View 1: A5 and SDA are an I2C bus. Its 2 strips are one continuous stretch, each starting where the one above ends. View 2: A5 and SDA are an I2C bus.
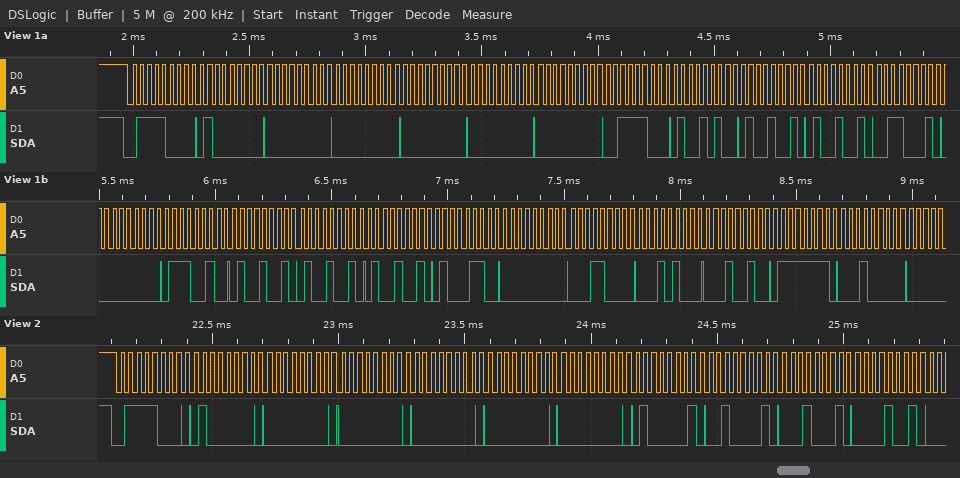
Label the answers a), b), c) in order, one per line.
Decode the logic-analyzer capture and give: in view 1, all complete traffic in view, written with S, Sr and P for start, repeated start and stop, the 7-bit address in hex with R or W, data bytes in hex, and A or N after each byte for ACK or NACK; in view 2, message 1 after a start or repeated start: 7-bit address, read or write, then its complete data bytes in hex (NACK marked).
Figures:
a) S 3CW A 40 A 00 A 00 A 00 A 00 A 00 A 3C A 4A A 49 A 49 A 31 A 00 A 72 A 49 A 49 A 49 A 46 A 00 A 18 A 14 A 12 A 7F A 10 A
b) 0x3C write: 40 00 00 00 00 00 41 21 11 09
